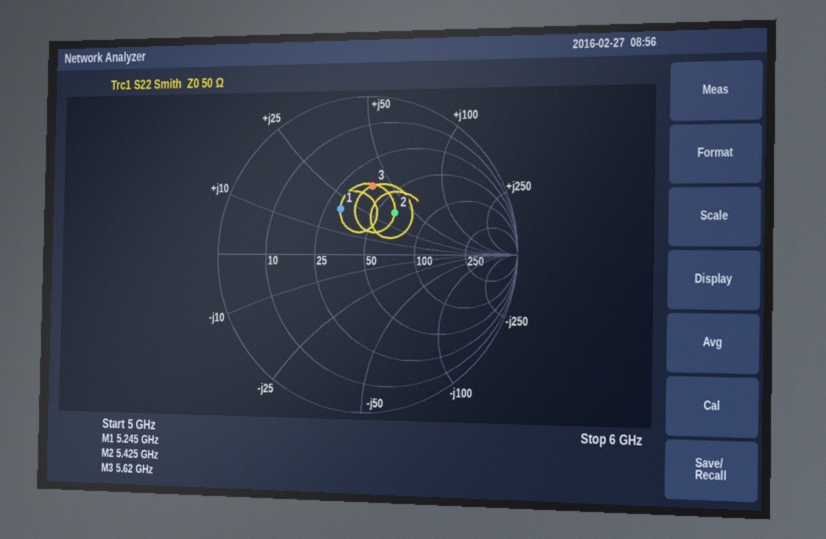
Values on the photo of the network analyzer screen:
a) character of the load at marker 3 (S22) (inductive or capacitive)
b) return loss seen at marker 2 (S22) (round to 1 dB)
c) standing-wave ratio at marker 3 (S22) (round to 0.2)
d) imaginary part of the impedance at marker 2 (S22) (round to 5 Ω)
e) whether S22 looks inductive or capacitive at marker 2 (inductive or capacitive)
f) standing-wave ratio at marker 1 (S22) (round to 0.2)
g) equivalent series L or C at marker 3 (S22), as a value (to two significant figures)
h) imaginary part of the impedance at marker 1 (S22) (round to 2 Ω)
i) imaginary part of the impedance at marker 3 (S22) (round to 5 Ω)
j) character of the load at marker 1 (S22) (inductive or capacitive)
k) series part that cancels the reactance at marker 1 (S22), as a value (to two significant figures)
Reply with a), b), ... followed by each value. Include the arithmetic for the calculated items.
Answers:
a) inductive
b) 10 dB
c) 2.6
d) +35 Ω
e) inductive
f) 2.0
g) L = 40 Ω/(2π × 5.62 GHz) ≈ 1.1 nH
h) +20 Ω
i) +40 Ω
j) inductive
k) C = 1/(2π × 5.245 GHz × 20 Ω) ≈ 1.5 pF
